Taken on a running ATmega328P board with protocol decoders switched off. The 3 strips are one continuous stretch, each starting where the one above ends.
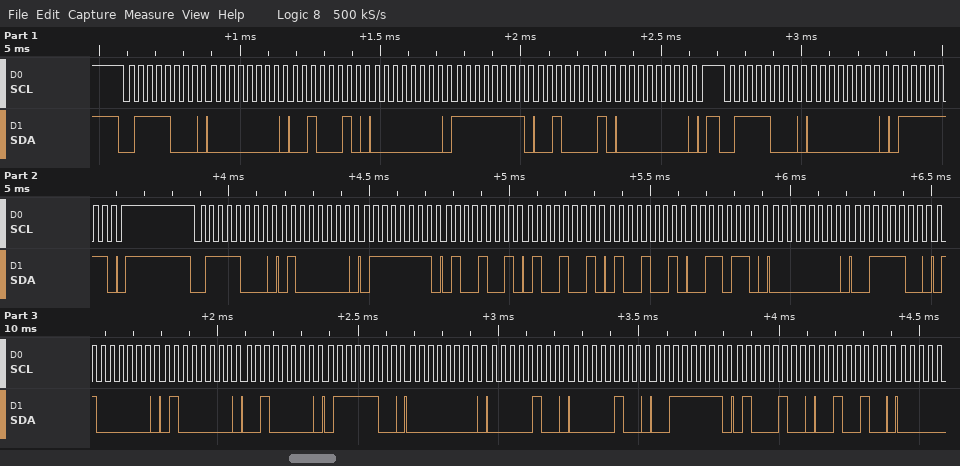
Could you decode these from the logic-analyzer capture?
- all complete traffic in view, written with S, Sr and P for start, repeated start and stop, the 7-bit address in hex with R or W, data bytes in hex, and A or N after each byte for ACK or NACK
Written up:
S 3CW A 00 A 22 A 00 A FF A 21 A 00 A P S 3CW A 00 A 7F A P S 3CW A 40 A 7F A 49 A 49 A 49 A 36 A 00 A 3C A 40 A 40 A 20 A 7C A 00 A 04 A 04 A 3F A 44 A 24 A
